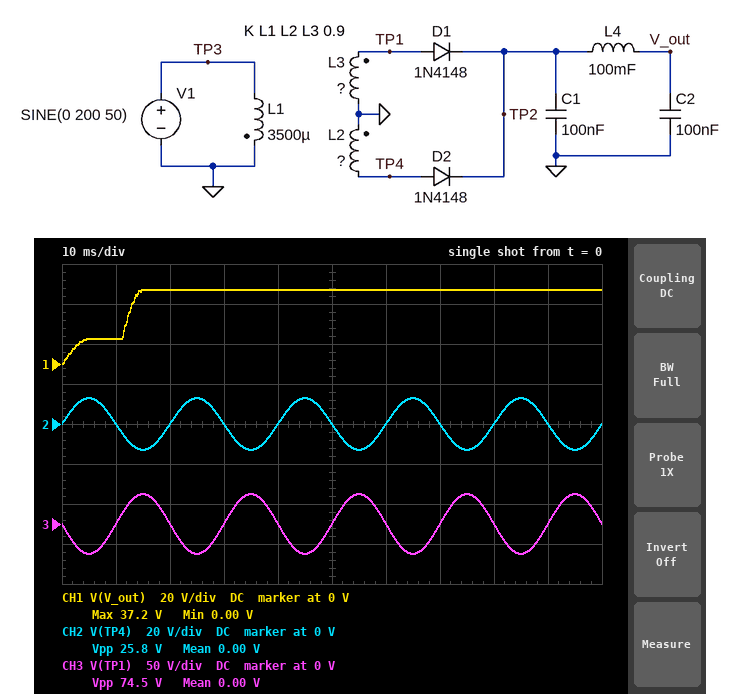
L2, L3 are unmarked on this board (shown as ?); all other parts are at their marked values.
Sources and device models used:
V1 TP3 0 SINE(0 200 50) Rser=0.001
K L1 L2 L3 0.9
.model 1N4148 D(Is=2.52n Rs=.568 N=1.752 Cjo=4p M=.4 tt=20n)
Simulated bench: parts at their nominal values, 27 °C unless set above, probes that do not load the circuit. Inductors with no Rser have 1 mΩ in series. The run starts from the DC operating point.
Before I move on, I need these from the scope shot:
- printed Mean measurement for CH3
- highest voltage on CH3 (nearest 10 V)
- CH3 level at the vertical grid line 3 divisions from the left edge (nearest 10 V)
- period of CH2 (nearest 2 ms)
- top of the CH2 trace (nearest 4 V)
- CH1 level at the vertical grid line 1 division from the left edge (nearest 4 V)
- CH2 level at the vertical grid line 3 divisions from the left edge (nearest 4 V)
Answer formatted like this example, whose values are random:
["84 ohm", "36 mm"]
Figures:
["0.00 V", "40 V", "0 V", "20 ms", "12 V", "12 V", "0 V"]
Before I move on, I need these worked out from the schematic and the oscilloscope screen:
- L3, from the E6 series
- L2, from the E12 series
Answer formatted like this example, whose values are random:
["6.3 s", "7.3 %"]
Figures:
["150 µH", "18 µH"]
